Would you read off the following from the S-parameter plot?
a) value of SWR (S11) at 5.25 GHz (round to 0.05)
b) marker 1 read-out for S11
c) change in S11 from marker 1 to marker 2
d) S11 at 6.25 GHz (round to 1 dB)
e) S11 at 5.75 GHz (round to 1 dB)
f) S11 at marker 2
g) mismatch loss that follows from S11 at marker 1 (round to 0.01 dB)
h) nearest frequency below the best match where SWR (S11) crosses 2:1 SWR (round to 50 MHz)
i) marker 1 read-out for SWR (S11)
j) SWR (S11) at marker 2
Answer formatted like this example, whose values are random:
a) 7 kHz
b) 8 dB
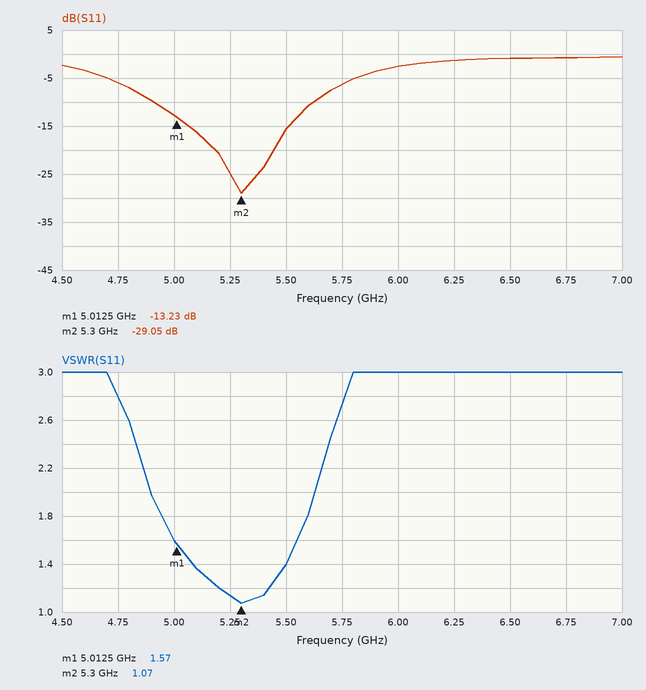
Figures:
a) 1.15
b) -13.23 dB
c) -15.82 dB
d) -1 dB
e) -6 dB
f) -29.05 dB
g) 0.21 dB
h) 4.90 GHz
i) 1.57
j) 1.07
